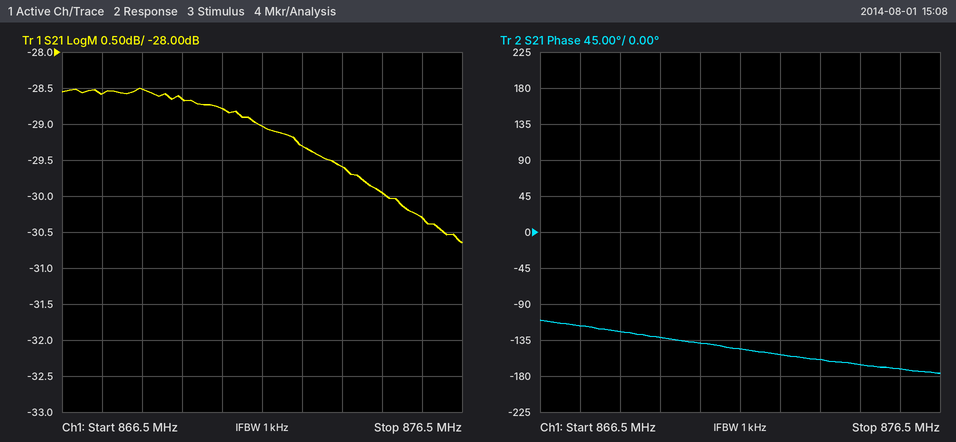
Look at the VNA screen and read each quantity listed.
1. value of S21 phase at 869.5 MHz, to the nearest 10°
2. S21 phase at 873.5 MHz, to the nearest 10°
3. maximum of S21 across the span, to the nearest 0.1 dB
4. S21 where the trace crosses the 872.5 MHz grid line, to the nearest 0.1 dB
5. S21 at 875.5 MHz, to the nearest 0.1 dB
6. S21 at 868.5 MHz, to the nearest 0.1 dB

-130°
-160°
-28.5 dB
-29.3 dB
-30.3 dB
-28.5 dB
